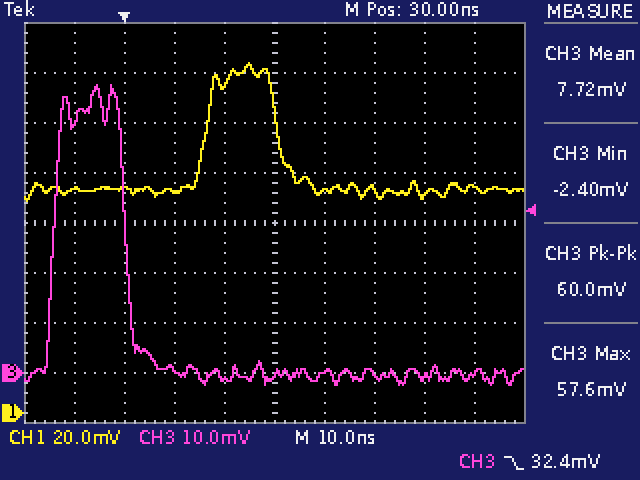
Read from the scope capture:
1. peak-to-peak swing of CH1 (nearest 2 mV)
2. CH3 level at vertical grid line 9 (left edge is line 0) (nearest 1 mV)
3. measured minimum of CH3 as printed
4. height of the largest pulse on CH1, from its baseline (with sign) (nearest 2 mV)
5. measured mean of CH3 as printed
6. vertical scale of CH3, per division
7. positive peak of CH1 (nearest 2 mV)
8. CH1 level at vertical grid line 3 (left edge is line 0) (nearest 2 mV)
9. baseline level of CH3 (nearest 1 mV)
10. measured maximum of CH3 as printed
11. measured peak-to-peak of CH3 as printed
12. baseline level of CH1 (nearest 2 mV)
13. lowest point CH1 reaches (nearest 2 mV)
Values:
56 mV
0 mV
-2.40 mV
+50 mV
7.72 mV
10 mV
140 mV
88 mV
0 mV
57.6 mV
60.0 mV
90 mV
84 mV
